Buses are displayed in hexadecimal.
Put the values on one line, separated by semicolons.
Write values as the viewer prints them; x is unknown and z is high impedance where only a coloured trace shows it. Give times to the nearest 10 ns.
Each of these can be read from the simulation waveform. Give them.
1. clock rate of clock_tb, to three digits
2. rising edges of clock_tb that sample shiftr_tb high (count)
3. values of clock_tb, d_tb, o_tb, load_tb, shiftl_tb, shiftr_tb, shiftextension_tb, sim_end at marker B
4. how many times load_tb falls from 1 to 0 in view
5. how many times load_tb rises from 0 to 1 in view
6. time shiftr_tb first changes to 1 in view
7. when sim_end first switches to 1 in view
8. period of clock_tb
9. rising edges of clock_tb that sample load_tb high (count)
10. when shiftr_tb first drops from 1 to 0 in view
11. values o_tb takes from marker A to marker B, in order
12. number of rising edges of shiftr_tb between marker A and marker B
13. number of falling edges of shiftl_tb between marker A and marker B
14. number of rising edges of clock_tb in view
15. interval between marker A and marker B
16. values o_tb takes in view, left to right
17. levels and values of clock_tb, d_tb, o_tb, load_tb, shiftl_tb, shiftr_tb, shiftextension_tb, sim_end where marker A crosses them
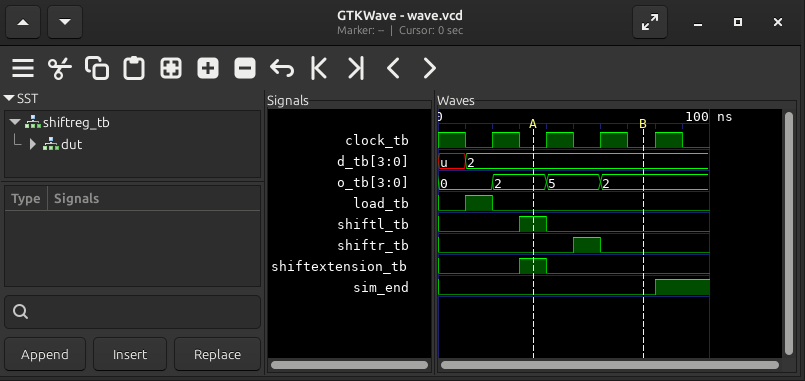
50.0 MHz; 1; clock_tb=0, d_tb=2, o_tb=2, load_tb=0, shiftl_tb=0, shiftr_tb=0, shiftextension_tb=0, sim_end=0; 1; 1; 50 ns; 80 ns; 20 ns; 1; 60 ns; 2, 5, 2; 1; 1; 4; 40 ns; 0, 2, 5, 2; clock_tb=0, d_tb=2, o_tb=2, load_tb=0, shiftl_tb=1, shiftr_tb=0, shiftextension_tb=1, sim_end=0
